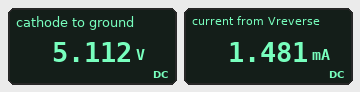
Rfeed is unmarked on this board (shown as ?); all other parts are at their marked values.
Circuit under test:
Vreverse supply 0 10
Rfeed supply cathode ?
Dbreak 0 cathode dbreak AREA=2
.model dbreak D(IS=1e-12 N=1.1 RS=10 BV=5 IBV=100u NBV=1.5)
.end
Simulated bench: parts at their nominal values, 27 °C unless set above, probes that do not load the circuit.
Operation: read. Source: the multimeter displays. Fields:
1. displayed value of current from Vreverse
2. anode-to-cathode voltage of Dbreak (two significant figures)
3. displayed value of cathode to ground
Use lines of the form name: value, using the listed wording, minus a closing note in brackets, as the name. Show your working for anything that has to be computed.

displayed value of current from Vreverse: 1.481 mA
anode-to-cathode voltage of Dbreak: 0 V - 5.112 V = -5.1 V
displayed value of cathode to ground: 5.112 V
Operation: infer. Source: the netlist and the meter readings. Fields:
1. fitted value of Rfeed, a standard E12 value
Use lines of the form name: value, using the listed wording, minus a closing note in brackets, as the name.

fitted value of Rfeed, a standard E12 value: 3.3 kΩ
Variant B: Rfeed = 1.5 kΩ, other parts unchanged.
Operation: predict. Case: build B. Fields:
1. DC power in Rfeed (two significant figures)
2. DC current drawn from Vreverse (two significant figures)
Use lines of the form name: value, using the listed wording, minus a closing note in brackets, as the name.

DC power in Rfeed: 16 mW
DC current drawn from Vreverse: 3.2 mA
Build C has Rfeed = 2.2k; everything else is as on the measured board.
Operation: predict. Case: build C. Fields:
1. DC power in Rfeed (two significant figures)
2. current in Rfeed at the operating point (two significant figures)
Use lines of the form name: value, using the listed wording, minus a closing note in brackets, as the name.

DC power in Rfeed: 11 mW
current in Rfeed at the operating point: 2.2 mA
